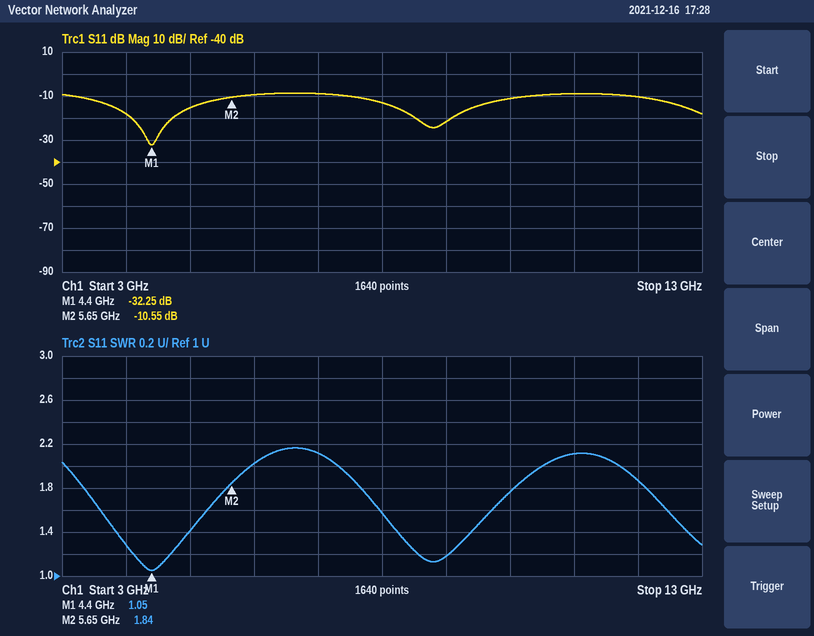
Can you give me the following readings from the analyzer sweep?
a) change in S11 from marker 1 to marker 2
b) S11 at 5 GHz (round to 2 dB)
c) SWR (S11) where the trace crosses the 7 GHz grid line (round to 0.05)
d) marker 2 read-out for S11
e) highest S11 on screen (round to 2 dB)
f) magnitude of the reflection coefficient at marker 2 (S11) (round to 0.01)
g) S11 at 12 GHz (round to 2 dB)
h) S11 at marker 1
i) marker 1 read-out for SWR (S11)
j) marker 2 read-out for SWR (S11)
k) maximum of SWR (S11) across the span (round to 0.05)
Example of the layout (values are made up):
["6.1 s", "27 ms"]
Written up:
["21.70 dB", "-16 dB", "2.10", "-10.55 dB", "-8 dB", "0.30", "-10 dB", "-32.25 dB", "1.05", "1.84", "2.15"]
